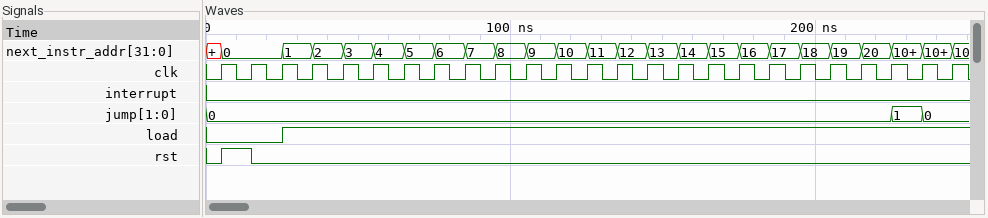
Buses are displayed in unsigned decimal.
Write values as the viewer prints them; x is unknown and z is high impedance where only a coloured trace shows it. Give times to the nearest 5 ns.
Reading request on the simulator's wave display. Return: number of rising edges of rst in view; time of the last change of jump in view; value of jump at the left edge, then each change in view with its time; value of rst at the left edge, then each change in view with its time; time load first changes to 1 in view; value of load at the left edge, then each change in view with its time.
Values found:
1
235 ns
0, 1 at 225 ns, 0 at 235 ns
0, 1 at 5 ns, 0 at 15 ns
25 ns
0, 1 at 25 ns
